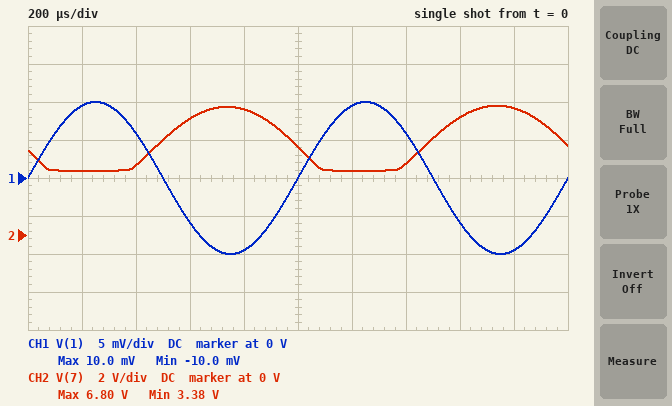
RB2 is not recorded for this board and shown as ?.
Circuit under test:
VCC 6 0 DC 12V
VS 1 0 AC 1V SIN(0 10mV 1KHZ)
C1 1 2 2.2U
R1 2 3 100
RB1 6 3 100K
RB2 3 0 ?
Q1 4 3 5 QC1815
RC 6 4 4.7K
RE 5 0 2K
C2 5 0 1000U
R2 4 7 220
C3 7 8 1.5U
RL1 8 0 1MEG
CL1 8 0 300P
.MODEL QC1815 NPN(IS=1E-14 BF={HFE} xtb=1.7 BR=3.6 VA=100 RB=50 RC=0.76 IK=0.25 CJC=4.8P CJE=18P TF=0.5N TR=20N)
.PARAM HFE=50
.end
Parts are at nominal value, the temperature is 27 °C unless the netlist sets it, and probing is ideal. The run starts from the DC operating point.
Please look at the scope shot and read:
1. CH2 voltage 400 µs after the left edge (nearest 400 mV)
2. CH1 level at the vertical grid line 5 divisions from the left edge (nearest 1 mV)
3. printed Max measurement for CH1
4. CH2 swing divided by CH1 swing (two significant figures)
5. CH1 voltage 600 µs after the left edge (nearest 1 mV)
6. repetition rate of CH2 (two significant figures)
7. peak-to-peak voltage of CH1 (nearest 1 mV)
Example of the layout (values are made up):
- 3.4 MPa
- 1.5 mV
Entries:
- 3.6 V
- 0 V
- 10.0 mV
- 170
- -6 mV
- 1.0 kHz
- 20 mV
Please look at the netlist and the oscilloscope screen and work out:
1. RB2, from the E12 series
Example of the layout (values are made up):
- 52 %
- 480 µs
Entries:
- 82 kΩ
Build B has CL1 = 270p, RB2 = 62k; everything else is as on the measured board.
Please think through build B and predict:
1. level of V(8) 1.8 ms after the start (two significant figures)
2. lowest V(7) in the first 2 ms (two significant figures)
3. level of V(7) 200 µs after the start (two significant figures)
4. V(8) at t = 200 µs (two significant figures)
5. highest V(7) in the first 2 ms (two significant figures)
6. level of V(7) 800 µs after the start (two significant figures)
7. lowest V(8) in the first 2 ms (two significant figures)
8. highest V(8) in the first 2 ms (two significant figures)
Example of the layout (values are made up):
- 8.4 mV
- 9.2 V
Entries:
- 1.8 V
- 3.3 V
- 3.4 V
- -2.0 V
- 7.3 V
- 7.2 V
- -2.1 V
- 1.9 V
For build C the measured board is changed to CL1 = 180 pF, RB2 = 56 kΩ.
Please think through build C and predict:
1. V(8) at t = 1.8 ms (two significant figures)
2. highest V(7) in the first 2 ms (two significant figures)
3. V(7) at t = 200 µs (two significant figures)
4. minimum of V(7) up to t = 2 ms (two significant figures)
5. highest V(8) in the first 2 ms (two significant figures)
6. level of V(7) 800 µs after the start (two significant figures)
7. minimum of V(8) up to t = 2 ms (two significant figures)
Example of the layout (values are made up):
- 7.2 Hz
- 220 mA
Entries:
- 1.7 V
- 7.6 V
- 3.8 V
- 3.7 V
- 1.8 V
- 7.5 V
- -2.0 V
